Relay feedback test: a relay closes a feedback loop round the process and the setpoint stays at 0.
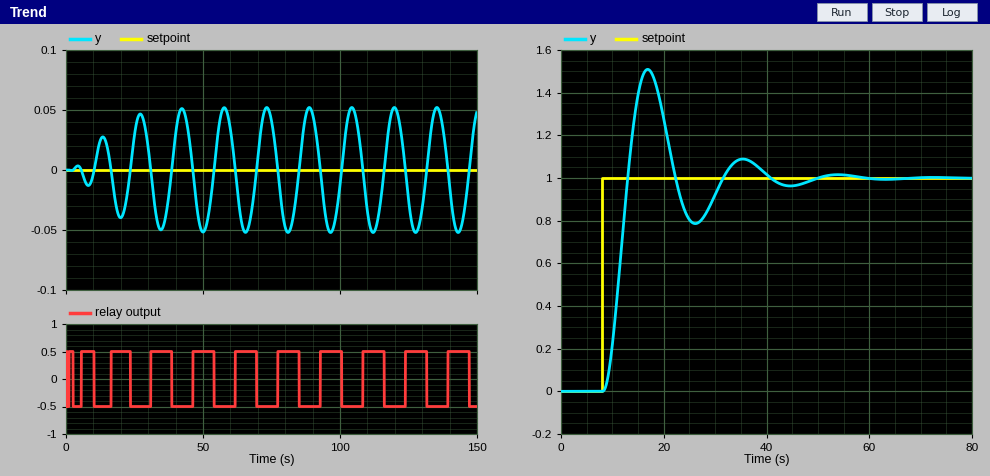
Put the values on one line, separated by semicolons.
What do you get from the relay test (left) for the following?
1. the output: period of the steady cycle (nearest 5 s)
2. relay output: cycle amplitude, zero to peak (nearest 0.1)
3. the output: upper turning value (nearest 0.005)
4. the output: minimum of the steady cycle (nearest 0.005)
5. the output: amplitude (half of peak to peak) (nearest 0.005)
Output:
15 s; 0.5; 0.050; -0.050; 0.050
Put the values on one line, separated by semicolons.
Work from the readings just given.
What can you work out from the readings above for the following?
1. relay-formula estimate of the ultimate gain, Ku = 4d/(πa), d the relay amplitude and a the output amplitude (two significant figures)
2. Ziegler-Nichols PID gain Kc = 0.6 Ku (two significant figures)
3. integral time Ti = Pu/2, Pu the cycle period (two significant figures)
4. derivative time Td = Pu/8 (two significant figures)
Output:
13; 7.8; 7.5 s; 1.9 s
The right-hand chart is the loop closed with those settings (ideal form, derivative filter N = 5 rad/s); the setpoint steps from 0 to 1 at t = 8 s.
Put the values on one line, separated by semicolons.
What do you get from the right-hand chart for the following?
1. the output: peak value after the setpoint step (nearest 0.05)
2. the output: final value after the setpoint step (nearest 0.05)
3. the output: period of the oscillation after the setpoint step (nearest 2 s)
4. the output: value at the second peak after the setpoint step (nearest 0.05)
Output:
1.50; 1.00; 18 s; 1.10
